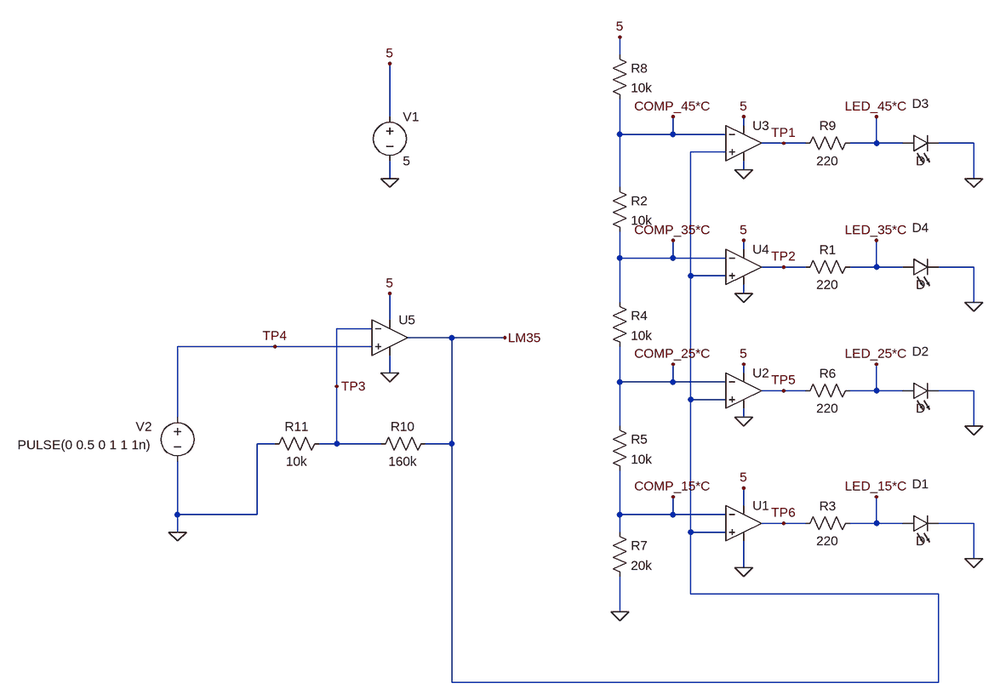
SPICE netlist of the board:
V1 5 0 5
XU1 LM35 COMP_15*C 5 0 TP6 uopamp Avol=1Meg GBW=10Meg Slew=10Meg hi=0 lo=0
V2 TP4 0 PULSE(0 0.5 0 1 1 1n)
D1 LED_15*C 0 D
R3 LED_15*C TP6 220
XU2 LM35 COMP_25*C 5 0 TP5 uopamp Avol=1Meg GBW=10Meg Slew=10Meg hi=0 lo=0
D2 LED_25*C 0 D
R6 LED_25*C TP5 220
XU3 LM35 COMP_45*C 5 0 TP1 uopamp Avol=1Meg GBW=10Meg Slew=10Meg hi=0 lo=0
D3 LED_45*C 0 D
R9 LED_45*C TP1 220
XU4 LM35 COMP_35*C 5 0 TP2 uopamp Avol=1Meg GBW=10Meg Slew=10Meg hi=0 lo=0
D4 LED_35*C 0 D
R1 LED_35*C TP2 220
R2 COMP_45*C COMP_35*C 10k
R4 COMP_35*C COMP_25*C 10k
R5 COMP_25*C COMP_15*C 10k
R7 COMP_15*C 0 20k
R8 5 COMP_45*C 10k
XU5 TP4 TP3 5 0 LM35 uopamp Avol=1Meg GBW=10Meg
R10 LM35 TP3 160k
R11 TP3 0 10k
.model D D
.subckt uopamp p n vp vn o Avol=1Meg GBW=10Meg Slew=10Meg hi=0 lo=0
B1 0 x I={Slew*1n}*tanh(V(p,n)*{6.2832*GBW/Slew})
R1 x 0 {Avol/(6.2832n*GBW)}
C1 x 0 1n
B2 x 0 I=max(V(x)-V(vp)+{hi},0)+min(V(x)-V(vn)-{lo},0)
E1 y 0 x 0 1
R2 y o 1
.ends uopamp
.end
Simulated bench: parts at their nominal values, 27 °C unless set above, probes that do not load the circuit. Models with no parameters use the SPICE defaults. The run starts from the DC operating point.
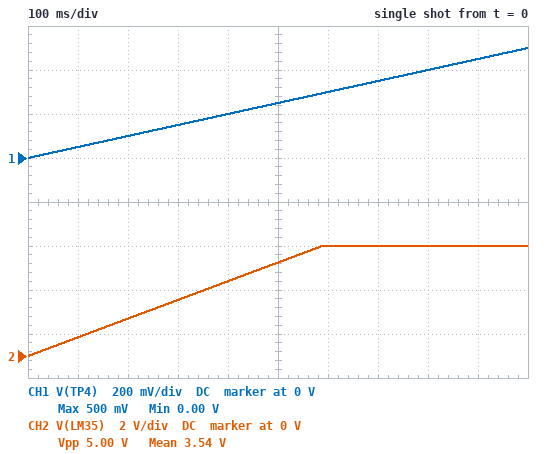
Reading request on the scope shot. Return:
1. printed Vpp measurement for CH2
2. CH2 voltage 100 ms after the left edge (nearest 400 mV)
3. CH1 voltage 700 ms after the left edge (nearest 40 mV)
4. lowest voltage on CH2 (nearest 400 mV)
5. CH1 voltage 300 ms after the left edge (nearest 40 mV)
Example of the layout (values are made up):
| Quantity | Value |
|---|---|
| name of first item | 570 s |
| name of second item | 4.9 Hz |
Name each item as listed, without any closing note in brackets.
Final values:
| Quantity | Value |
|---|---|
| printed Vpp measurement for CH2 | 5.00 V |
| CH2 voltage 100 ms after the left edge | 800 mV |
| CH1 voltage 700 ms after the left edge | 360 mV |
| lowest voltage on CH2 | 0 V |
| CH1 voltage 300 ms after the left edge | 160 mV |
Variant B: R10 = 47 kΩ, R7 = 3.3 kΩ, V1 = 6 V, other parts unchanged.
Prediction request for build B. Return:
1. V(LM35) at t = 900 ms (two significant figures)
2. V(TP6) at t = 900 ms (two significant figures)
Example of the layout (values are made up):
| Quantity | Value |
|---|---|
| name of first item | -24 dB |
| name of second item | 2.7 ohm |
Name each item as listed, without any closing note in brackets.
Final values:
| Quantity | Value |
|---|---|
| V(LM35) at t = 900 ms | 2.6 V |
| V(TP6) at t = 900 ms | 6.0 V |
